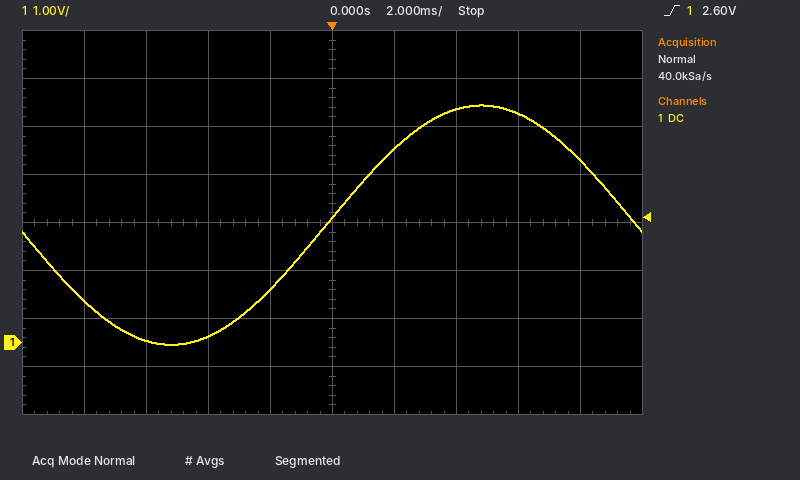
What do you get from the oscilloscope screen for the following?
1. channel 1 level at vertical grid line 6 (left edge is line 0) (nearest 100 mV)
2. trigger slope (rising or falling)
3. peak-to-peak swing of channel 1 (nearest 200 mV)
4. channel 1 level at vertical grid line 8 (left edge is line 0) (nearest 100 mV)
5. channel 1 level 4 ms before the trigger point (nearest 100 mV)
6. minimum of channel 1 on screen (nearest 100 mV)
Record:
4.0 V
rising
5.0 V
4.8 V
100 mV
0.0 V
